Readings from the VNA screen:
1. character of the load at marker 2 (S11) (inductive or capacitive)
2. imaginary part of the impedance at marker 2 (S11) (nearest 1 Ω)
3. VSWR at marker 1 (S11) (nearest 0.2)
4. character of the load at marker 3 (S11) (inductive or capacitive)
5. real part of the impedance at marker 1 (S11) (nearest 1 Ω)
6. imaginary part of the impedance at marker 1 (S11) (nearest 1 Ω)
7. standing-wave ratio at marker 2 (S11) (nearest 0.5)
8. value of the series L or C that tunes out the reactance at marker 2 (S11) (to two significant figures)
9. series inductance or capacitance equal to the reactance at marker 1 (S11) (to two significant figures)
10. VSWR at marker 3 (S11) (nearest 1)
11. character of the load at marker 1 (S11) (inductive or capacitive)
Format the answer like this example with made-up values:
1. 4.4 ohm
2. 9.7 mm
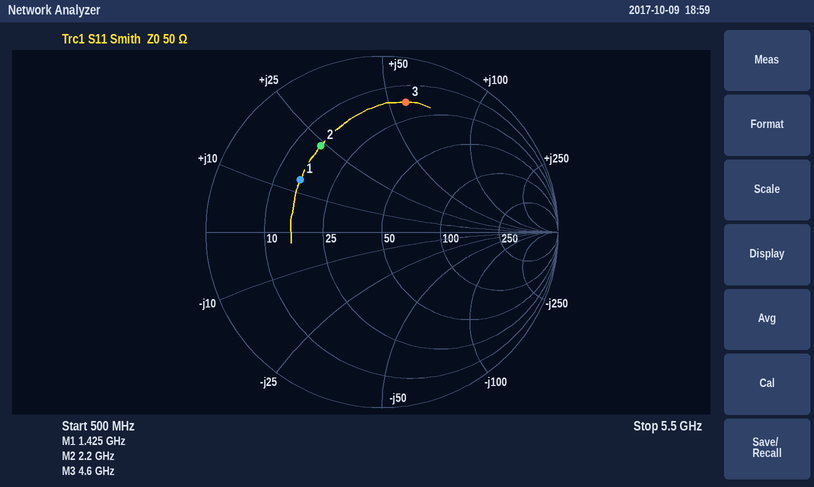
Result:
1. inductive
2. +24 Ω
3. 3.4
4. inductive
5. 16 Ω
6. +13 Ω
7. 4.0
8. 3.0 pF
9. 1.5 nH
10. 7
11. inductive
